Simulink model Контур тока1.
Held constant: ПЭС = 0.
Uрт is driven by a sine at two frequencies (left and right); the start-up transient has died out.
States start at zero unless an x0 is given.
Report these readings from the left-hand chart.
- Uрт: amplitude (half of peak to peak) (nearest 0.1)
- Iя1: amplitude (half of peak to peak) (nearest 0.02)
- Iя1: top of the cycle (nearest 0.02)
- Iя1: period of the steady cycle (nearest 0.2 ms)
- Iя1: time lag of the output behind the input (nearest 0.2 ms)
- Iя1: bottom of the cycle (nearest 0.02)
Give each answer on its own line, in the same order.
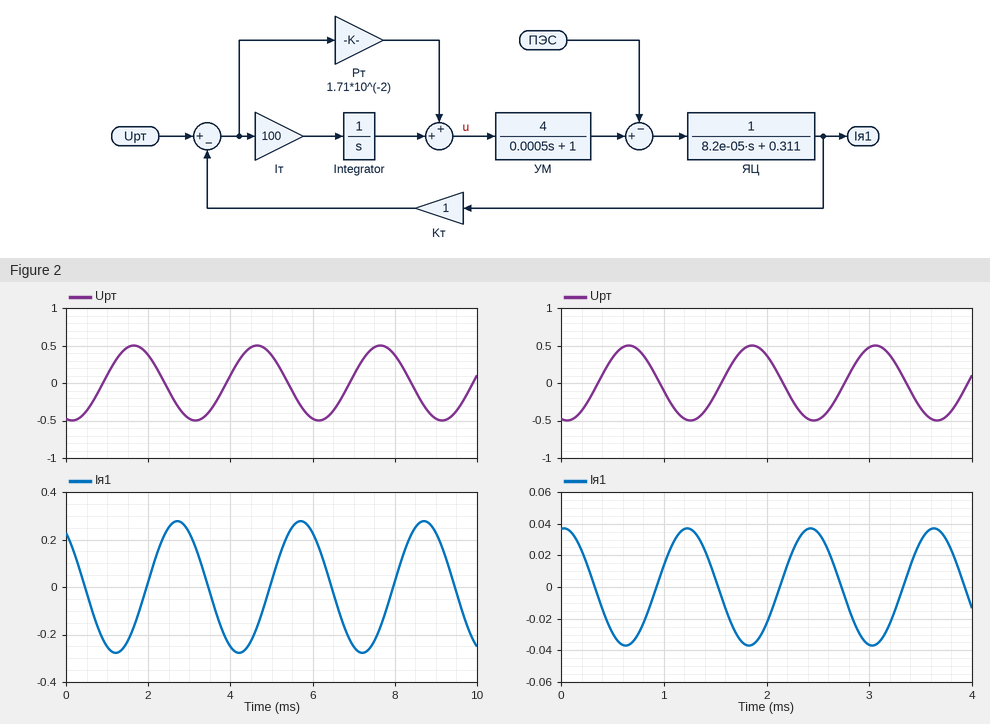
0.5
0.28
0.28
3.0 ms
1.0 ms
-0.28
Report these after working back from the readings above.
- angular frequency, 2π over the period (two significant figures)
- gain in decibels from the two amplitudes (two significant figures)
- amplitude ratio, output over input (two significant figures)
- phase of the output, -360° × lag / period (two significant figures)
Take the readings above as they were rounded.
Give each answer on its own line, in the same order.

2.1 rad/ms
-5.0 dB
0.56
-120°
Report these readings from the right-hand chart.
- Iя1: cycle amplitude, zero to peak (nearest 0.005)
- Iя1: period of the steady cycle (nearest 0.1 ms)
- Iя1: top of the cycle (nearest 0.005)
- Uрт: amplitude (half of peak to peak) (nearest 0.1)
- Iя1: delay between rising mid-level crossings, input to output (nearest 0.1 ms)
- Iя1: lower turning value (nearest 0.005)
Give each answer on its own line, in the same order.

0.035
1.2 ms
0.035
0.5
0.6 ms
-0.035
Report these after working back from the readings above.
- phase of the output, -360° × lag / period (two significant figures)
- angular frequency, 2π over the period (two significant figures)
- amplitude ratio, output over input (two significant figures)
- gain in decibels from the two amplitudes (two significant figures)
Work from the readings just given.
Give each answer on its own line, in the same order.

-180°
5.2 rad/ms
0.070
-23 dB
